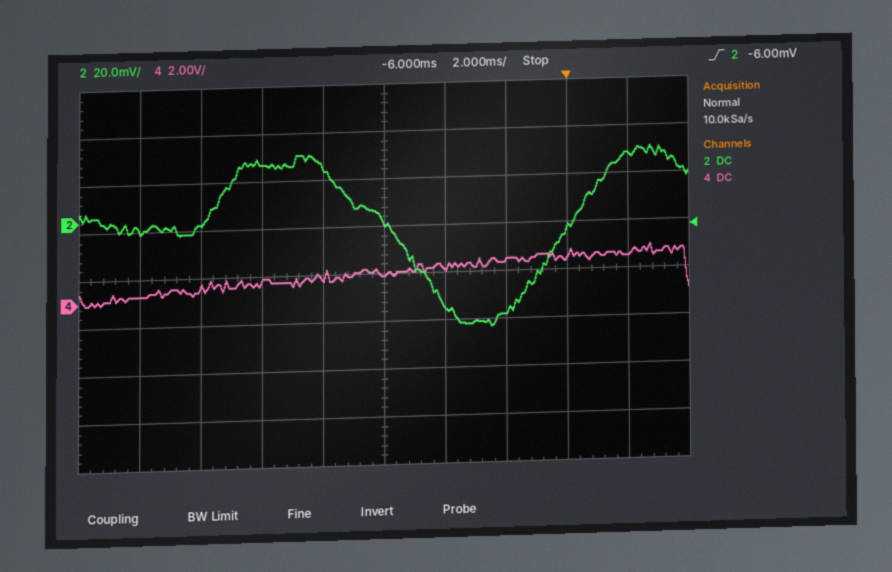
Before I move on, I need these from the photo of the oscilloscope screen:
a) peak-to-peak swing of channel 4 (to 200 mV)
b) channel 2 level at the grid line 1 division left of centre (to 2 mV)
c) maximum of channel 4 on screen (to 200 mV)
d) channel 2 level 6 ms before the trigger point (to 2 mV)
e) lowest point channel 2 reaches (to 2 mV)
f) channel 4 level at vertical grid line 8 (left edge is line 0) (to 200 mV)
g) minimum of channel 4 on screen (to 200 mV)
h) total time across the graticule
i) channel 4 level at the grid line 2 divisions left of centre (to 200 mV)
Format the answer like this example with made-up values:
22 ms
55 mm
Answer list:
2.0 V
22 mV
2.0 V
-2 mV
-46 mV
1.6 V
0.0 V
20 ms
800 mV
